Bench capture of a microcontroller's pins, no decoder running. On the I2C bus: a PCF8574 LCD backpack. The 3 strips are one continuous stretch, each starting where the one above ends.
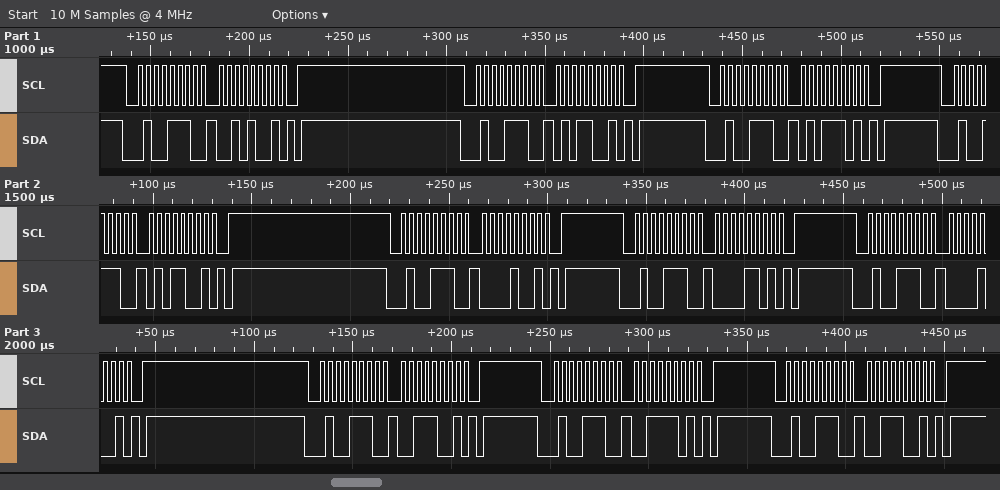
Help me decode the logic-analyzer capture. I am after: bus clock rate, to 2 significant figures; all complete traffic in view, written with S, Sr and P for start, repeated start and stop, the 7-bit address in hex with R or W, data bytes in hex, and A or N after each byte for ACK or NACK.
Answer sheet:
250 kHz
S 27W A 29 A P S 27W A 59 A P S 27W A 5D A P S 27W A 59 A P S 27W A 09 A P S 27W A 0D A P S 27W A 09 A P S 27W A 39 A P S 27W A 3D A P S 27W A 39 A P
